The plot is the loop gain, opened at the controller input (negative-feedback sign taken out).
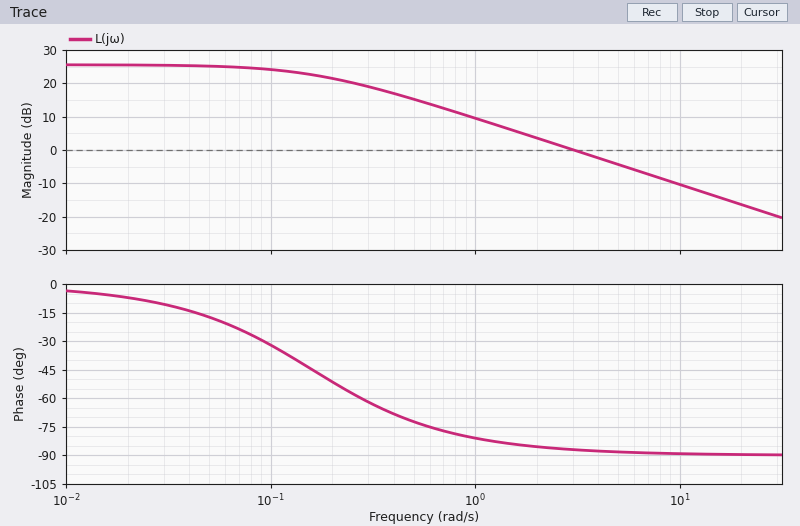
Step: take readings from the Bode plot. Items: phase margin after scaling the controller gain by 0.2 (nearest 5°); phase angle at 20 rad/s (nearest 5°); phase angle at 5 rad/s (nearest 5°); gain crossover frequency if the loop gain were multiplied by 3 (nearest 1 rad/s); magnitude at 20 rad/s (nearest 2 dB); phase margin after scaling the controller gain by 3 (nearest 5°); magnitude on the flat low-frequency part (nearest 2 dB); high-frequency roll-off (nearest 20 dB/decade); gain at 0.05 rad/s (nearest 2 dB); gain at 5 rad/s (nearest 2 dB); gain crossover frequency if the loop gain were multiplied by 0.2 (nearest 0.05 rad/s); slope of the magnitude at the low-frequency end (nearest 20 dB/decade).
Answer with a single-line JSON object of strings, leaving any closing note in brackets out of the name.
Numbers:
{"phase margin after scaling the controller gain by 0.2": "105°", "phase angle at 20 rad/s": "-90°", "phase angle at 5 rad/s": "-90°", "gain crossover frequency if the loop gain were multiplied by 3": "9 rad/s", "magnitude at 20 rad/s": "-16 dB", "phase margin after scaling the controller gain by 3": "90°", "magnitude on the flat low-frequency part": "26 dB", "high-frequency roll-off": "-20 dB/decade", "gain at 0.05 rad/s": "26 dB", "gain at 5 rad/s": "-4 dB", "gain crossover frequency if the loop gain were multiplied by 0.2": "0.60 rad/s", "slope of the magnitude at the low-frequency end": "0 dB/decade"}
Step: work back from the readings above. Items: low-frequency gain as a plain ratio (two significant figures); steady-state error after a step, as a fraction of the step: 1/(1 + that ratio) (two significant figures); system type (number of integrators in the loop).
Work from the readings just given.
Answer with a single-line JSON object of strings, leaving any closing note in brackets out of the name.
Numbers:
{"low-frequency gain as a plain ratio": "20", "steady-state error after a step, as a fraction of the step: 1/(1 + that ratio)": "0.048", "system type": "0"}
